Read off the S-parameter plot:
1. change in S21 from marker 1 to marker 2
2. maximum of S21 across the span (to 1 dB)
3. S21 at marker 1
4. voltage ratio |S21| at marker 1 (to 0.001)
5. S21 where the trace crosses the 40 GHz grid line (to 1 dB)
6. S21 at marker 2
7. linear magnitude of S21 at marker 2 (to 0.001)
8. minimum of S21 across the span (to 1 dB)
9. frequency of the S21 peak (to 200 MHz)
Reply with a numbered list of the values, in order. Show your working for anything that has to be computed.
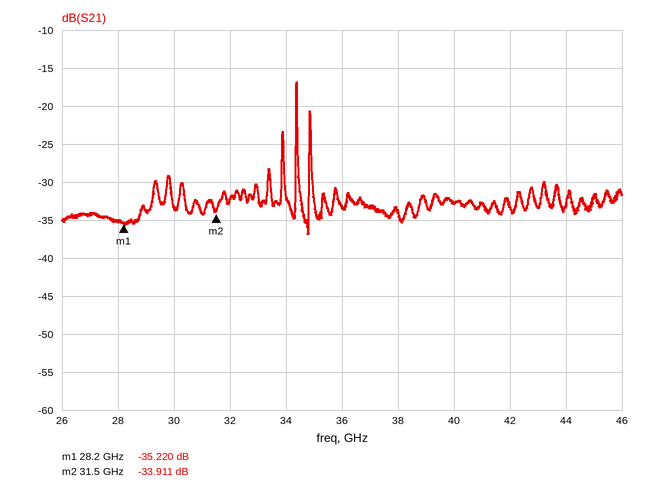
1. -33.911 − (-35.22) = 1.309 dB
2. -17 dB
3. -35.220 dB
4. 10^(-35.22/20) ≈ 0.017
5. -33 dB
6. -33.911 dB
7. 10^(-33.911/20) ≈ 0.020
8. -37 dB
9. 34.4 GHz
